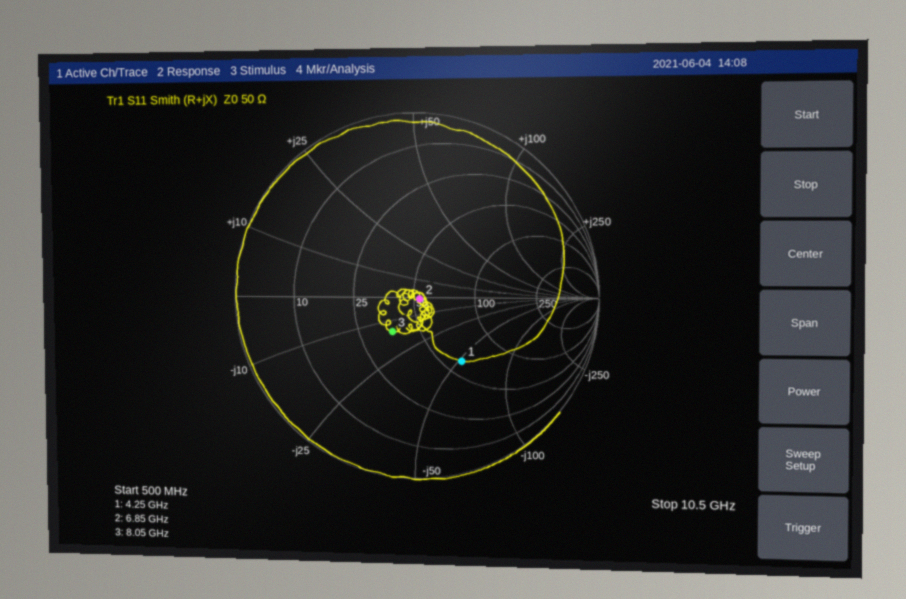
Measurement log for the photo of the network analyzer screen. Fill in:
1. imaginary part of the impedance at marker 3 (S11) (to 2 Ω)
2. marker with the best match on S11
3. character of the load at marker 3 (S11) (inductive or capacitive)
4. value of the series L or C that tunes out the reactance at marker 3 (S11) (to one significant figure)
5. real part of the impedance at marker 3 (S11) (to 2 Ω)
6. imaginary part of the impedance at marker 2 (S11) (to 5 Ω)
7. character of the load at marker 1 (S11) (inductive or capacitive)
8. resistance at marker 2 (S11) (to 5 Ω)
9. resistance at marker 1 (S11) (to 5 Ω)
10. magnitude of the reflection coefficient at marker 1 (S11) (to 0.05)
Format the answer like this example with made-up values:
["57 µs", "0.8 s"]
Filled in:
["-14 Ω", "marker 2", "capacitive", "300 pH", "36 Ω", "0 Ω", "capacitive", "55 Ω", "60 Ω", "0.45"]
